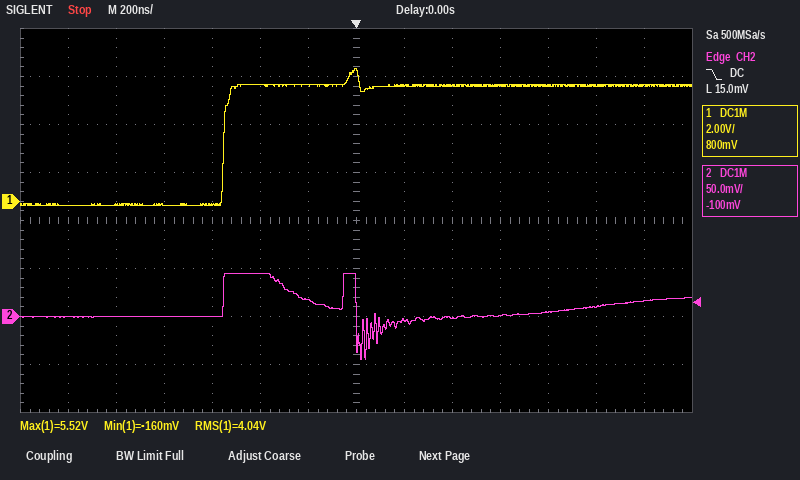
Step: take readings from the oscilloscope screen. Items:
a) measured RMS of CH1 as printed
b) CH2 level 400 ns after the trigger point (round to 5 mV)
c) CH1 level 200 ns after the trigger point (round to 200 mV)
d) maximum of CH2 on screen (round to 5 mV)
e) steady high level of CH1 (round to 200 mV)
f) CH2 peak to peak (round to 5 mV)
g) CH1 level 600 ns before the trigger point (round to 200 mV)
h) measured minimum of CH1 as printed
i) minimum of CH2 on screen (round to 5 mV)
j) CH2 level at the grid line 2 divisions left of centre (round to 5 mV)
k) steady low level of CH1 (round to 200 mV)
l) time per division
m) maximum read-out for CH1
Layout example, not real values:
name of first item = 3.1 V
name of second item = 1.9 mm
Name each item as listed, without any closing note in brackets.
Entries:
measured RMS of CH1 as printed = 4.04 V
CH2 level 400 ns after the trigger point = 0 mV
CH1 level 200 ns after the trigger point = 4.8 V
maximum of CH2 on screen = 45 mV
steady high level of CH1 = 4.8 V
CH2 peak to peak = 90 mV
CH1 level 600 ns before the trigger point = -200 mV
measured minimum of CH1 as printed = -160 mV
minimum of CH2 on screen = -45 mV
CH2 level at the grid line 2 divisions left of centre = 45 mV
steady low level of CH1 = -200 mV
time per division = 200 ns
maximum read-out for CH1 = 5.52 V
